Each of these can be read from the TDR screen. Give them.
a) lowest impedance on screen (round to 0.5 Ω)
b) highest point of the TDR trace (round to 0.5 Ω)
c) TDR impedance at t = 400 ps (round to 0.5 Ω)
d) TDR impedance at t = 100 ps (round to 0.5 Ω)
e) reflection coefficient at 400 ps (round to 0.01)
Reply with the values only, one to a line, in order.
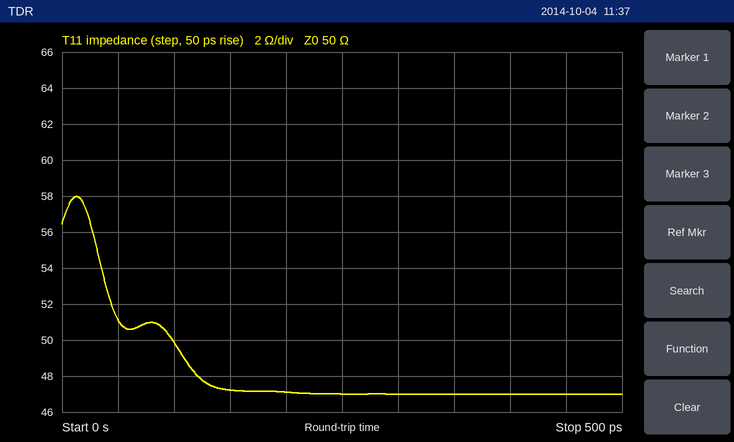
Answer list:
47.0 Ω
58.0 Ω
47.0 Ω
50.0 Ω
-0.03
